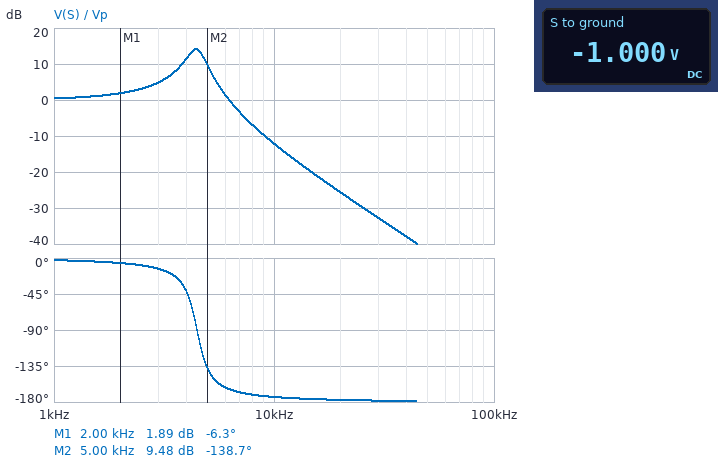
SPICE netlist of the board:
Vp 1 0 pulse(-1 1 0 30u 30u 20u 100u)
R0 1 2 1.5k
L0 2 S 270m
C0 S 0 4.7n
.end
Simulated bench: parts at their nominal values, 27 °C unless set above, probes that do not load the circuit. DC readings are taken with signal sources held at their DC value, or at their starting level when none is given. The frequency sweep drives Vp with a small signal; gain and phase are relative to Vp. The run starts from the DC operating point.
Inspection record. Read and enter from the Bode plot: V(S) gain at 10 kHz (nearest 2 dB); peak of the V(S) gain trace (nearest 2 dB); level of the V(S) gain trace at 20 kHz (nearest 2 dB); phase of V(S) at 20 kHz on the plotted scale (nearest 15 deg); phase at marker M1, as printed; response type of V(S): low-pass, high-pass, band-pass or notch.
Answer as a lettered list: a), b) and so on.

a) -12 dB
b) 14 dB
c) -26 dB
d) -180 deg
e) -6.3 deg
f) low-pass
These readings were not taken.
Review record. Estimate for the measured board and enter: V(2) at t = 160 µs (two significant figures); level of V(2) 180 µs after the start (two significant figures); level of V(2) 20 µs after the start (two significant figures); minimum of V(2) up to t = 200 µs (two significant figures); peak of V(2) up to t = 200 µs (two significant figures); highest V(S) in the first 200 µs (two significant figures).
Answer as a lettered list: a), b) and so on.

a) 370 mV
b) -940 mV
c) 260 mV
d) -1.2 V
e) 1.2 V
f) 1.2 V
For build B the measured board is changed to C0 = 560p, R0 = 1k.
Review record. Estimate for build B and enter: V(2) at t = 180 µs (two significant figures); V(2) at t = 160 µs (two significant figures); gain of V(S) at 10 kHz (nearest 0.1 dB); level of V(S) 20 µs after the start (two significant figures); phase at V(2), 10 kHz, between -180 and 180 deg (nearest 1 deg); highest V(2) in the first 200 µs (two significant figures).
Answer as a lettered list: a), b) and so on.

a) -920 mV
b) 470 mV
c) 7.9 dB
d) -490 mV
e) -5 deg
f) 1.1 V
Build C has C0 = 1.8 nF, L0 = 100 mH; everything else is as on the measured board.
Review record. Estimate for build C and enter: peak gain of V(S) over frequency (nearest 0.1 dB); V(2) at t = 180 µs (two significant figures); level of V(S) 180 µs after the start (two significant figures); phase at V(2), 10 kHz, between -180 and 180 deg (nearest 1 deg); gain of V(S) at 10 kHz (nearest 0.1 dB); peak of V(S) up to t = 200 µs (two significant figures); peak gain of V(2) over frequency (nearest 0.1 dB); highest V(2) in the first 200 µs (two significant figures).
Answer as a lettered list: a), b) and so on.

a) 14.0 dB
b) -400 mV
c) -900 mV
d) -30 deg
e) 9.5 dB
f) 3.4 V
g) 0 dB
h) 920 mV
